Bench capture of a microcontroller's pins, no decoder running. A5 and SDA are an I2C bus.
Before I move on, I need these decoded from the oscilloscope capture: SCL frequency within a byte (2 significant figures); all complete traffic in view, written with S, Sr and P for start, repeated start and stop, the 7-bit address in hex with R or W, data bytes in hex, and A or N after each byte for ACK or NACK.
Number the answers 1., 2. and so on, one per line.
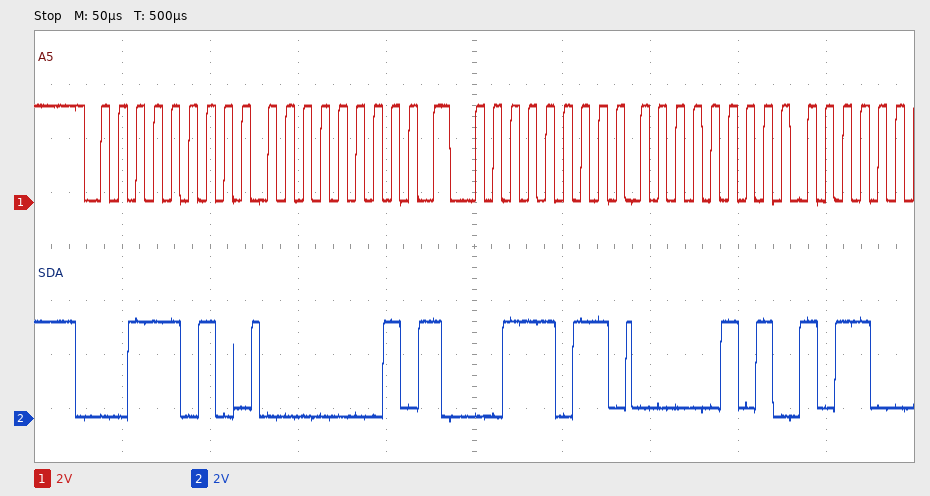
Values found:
1. 100 kHz
2. S 1DW A 01 A Sr 1DR A 05 A
